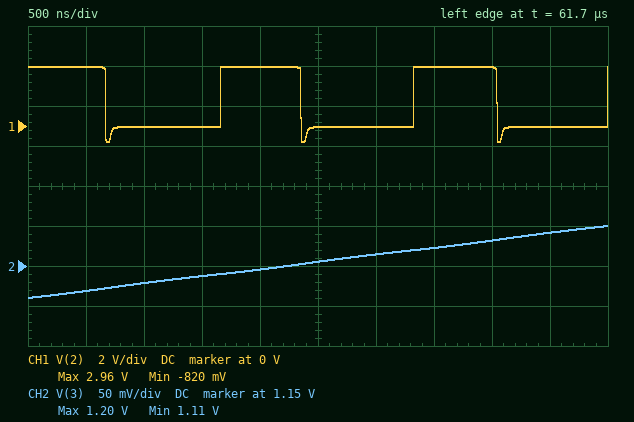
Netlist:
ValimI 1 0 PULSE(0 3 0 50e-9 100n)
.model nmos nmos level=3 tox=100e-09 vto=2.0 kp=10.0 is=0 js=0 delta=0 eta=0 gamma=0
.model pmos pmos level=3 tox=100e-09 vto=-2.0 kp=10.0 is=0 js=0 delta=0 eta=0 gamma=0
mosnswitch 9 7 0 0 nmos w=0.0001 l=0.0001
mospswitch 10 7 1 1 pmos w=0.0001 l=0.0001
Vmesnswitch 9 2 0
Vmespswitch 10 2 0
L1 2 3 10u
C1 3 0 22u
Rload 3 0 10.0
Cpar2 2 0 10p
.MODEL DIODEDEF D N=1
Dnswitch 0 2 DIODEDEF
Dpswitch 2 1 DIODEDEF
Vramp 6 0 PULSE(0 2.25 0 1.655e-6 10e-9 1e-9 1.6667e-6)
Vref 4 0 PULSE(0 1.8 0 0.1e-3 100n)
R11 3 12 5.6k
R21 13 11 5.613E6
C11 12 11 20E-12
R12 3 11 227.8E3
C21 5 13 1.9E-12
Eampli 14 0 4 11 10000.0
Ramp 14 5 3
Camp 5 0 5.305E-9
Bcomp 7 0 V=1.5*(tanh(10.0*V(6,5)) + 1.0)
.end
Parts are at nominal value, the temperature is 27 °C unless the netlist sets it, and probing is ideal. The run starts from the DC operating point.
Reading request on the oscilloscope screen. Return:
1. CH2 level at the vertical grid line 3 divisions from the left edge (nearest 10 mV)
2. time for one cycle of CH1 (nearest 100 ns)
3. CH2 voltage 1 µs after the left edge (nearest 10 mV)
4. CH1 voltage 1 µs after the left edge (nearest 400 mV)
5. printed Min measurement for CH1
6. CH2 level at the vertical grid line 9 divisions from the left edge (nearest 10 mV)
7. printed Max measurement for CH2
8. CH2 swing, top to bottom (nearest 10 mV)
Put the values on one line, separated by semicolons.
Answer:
1.14 V; 1.7 µs; 1.13 V; 0 V; -820 mV; 1.19 V; 1.20 V; 90 mV
